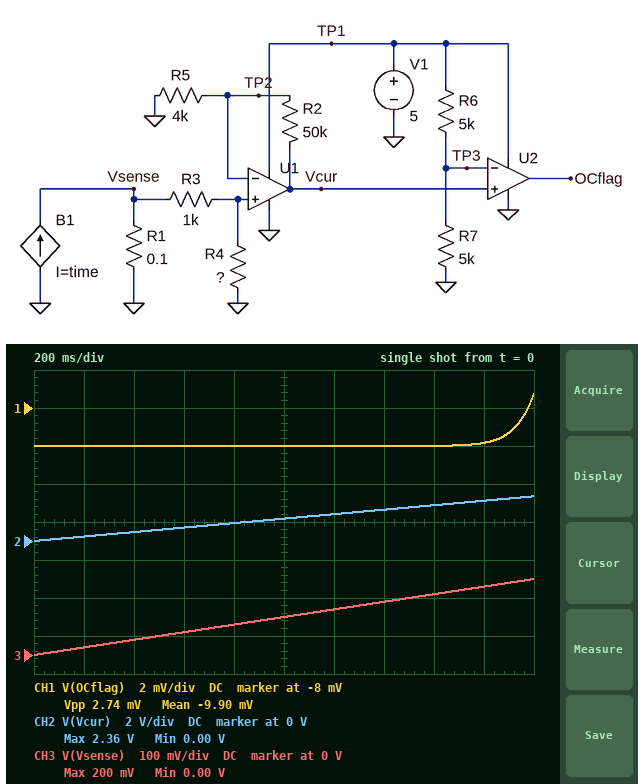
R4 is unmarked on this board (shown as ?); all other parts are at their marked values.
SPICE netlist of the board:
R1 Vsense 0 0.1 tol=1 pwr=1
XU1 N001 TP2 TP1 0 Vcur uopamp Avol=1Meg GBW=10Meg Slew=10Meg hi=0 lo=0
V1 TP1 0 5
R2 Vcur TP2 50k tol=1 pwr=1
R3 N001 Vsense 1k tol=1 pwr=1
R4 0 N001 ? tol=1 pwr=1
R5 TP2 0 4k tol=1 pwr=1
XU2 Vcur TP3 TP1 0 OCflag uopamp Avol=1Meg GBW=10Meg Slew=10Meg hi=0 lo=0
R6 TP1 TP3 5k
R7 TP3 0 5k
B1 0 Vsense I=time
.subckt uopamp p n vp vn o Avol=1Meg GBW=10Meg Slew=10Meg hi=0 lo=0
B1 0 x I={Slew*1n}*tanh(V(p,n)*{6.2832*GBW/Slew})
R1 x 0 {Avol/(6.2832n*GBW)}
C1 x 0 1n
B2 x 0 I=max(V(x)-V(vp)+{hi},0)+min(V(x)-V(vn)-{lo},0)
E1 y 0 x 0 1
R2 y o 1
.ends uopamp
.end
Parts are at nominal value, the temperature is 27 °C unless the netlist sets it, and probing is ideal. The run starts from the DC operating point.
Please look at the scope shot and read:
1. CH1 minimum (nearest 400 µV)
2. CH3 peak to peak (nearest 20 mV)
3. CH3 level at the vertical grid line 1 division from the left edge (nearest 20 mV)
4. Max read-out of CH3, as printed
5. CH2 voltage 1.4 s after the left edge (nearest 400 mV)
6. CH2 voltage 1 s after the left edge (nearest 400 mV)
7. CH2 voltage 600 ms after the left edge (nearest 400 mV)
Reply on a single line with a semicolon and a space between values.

-10.0 mV; 200 mV; 20 mV; 200 mV; 1.6 V; 1.2 V; 800 mV
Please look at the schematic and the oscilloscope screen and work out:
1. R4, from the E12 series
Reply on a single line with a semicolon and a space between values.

6.8 kΩ
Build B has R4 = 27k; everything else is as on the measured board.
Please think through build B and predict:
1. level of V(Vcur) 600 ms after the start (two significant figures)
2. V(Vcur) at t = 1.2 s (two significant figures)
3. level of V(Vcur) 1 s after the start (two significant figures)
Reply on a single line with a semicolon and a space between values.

780 mV; 1.6 V; 1.3 V
